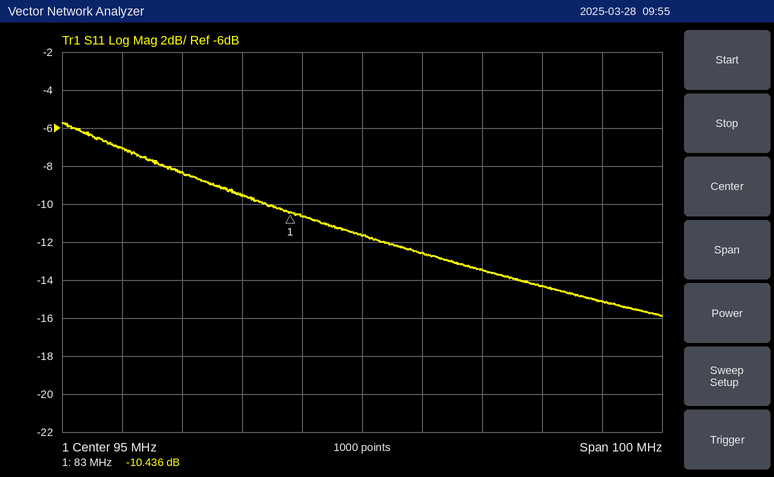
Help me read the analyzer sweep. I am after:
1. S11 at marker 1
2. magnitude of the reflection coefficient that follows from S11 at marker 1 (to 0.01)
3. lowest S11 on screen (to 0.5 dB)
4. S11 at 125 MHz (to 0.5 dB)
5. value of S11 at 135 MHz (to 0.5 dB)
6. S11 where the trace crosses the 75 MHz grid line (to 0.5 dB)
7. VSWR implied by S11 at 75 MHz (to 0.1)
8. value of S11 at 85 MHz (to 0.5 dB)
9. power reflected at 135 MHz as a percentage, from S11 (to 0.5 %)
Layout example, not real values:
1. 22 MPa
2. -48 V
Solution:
1. -10.436 dB
2. 0.30
3. -16.0 dB
4. -14.5 dB
5. -15.0 dB
6. -9.5 dB
7. 2.0
8. -10.5 dB
9. 3.0 %
